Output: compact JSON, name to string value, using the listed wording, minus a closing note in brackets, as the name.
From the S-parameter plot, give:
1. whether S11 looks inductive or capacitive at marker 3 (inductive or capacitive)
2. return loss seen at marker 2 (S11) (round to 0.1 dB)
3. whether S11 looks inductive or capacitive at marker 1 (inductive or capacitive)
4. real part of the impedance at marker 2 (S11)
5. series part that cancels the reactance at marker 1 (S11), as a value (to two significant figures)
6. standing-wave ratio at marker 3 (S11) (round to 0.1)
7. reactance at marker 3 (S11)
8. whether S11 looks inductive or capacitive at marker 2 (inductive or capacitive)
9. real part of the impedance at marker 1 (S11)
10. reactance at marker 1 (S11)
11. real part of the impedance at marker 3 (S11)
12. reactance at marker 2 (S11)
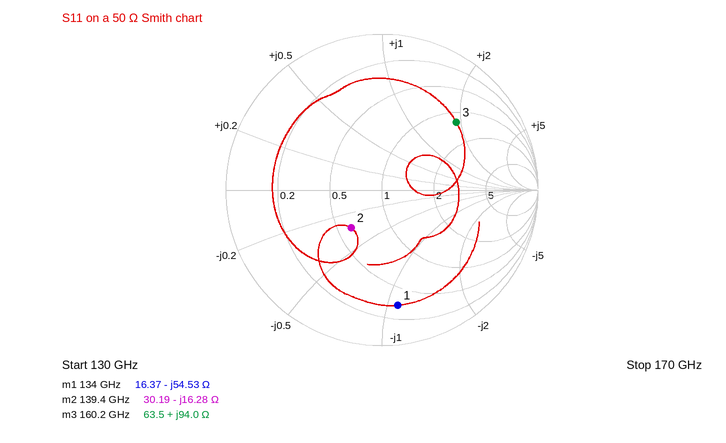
{"whether S11 looks inductive or capacitive at marker 3": "inductive", "return loss seen at marker 2 (S11)": "10.1 dB", "whether S11 looks inductive or capacitive at marker 1": "capacitive", "real part of the impedance at marker 2": "30.19 Ω", "series part that cancels the reactance at marker 1 (S11), as a value": "65 pH", "standing-wave ratio at marker 3 (S11)": "4.6", "reactance at marker 3": "+94.0 Ω", "whether S11 looks inductive or capacitive at marker 2": "capacitive", "real part of the impedance at marker 1": "16.37 Ω", "reactance at marker 1": "-54.53 Ω", "real part of the impedance at marker 3": "63.5 Ω", "reactance at marker 2": "-16.28 Ω"}
